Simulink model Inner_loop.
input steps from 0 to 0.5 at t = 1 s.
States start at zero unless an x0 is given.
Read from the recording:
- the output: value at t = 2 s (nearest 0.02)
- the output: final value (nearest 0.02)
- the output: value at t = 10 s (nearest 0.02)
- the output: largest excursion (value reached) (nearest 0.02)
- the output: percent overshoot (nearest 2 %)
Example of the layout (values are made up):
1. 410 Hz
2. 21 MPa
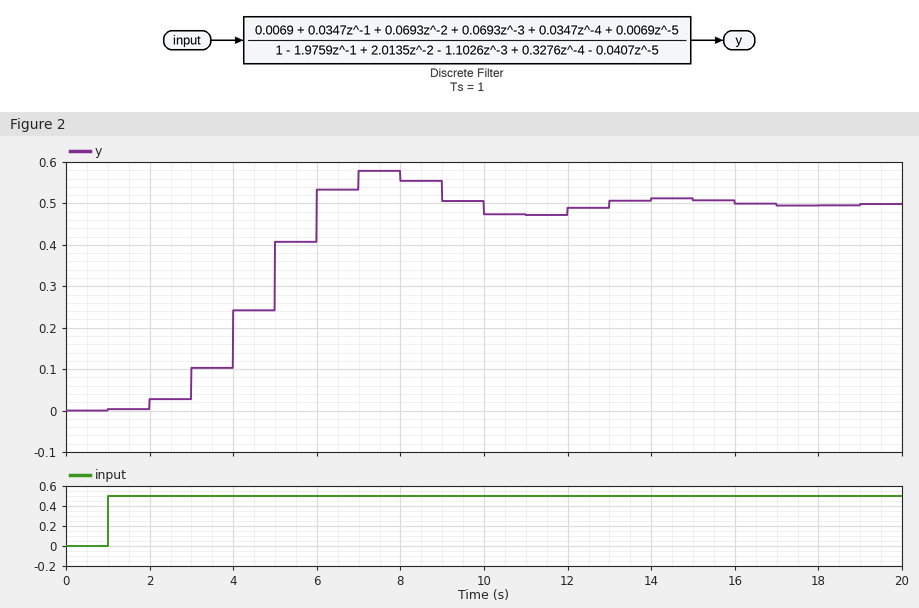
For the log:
1. 0.02
2. 0.50
3. 0.48
4. 0.58
5. 16 %
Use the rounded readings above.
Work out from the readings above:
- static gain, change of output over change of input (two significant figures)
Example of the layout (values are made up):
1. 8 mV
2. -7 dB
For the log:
1. 1.0
